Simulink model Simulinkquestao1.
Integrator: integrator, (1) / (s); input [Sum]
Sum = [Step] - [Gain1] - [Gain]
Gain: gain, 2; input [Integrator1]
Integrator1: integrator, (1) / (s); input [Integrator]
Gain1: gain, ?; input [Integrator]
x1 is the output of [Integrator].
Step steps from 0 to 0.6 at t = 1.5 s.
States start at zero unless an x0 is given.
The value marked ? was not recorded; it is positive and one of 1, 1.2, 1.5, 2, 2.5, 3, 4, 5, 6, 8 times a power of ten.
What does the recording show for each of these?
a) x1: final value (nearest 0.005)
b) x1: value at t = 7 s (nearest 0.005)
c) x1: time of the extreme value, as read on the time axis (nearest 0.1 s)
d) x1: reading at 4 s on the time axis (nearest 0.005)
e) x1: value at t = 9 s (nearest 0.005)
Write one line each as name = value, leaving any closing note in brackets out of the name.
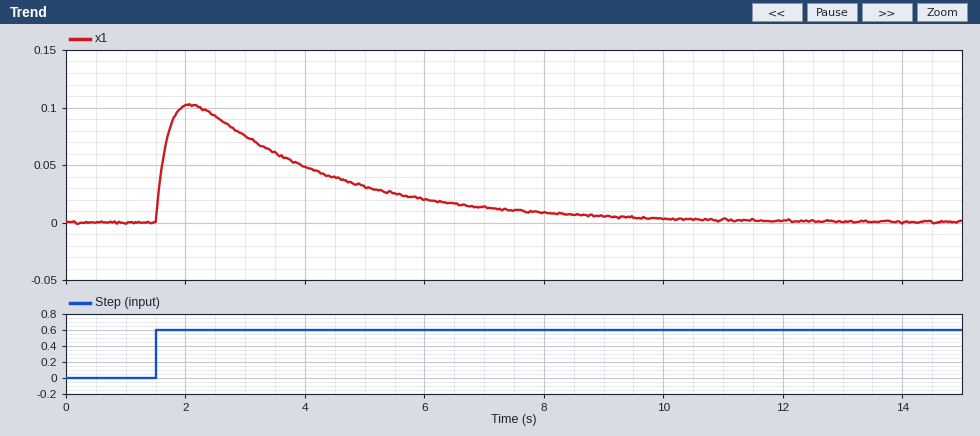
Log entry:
x1: final value = 0.000
x1: value at t = 7 s = 0.015
x1: time of the extreme value, as read on the time axis = 2.1 s
x1: reading at 4 s on the time axis = 0.050
x1: value at t = 9 s = 0.005
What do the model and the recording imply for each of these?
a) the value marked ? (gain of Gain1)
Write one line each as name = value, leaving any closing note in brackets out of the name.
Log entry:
the value marked ? = 5
